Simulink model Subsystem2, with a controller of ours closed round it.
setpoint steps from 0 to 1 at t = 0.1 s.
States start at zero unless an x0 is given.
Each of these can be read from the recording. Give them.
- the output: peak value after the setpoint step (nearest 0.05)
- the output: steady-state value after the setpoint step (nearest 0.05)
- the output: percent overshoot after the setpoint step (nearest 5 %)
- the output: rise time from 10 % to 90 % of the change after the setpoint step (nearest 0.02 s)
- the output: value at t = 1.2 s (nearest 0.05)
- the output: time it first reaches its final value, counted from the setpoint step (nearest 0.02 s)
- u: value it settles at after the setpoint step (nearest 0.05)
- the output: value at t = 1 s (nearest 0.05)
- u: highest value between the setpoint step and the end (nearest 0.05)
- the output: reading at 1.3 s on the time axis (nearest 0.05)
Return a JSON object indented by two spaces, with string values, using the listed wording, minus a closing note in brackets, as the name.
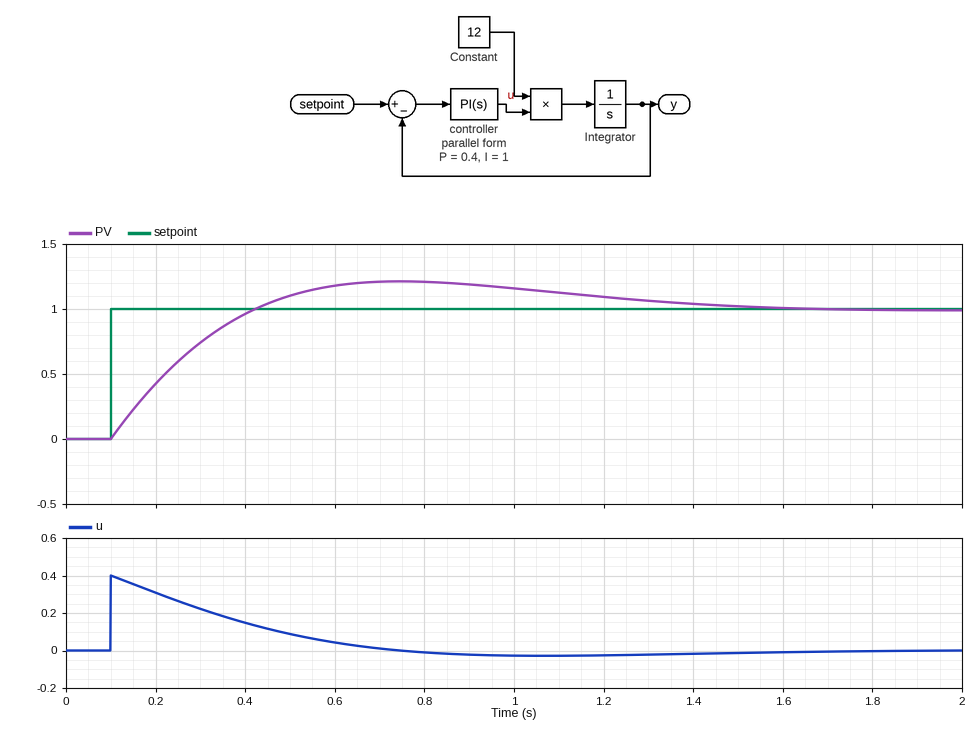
{
  "the output: peak value after the setpoint step": "1.20",
  "the output: steady-state value after the setpoint step": "1.00",
  "the output: percent overshoot after the setpoint step": "20 %",
  "the output: rise time from 10 % to 90 % of the change after the setpoint step": "0.24 s",
  "the output: value at t = 1.2 s": "1.10",
  "the output: time it first reaches its final value, counted from the setpoint step": "0.32 s",
  "u: value it settles at after the setpoint step": "0.00",
  "the output: value at t = 1 s": "1.15",
  "u: highest value between the setpoint step and the end": "0.40",
  "the output: reading at 1.3 s on the time axis": "1.05"
}
